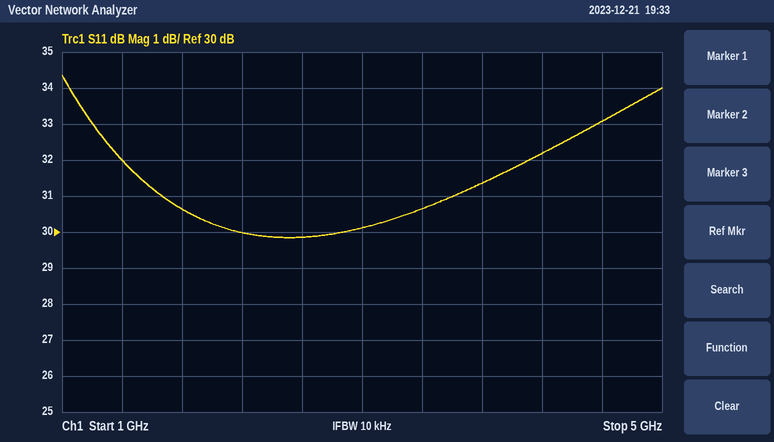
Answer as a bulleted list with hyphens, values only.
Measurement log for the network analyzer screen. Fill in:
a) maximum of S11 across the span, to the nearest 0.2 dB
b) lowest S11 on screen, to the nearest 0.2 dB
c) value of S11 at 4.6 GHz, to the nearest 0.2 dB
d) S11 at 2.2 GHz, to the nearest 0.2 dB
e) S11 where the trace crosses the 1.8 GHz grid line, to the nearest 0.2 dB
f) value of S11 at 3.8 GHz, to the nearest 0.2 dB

- 34.4 dB
- 29.8 dB
- 33.0 dB
- 30.0 dB
- 30.6 dB
- 31.4 dB
